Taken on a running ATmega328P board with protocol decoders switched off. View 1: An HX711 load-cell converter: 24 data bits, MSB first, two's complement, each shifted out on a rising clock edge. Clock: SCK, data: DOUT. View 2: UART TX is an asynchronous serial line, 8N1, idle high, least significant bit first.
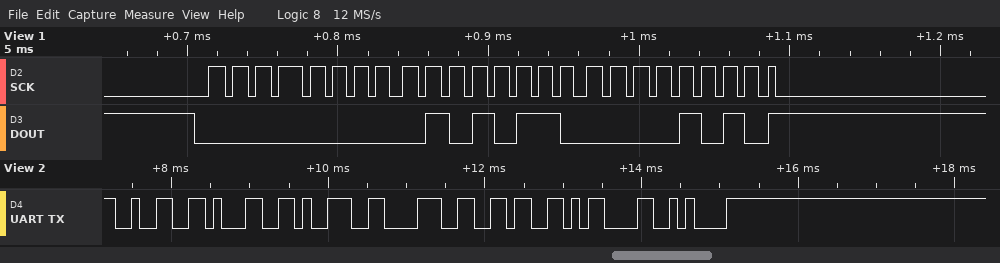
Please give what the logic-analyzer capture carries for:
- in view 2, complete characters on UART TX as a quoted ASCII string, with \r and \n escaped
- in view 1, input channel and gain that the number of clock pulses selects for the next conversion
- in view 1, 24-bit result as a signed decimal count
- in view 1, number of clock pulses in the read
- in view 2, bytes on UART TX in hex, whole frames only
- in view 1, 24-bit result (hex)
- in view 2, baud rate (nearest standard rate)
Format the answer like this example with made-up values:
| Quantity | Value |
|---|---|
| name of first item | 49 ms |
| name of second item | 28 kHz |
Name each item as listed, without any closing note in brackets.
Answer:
| Quantity | Value |
|---|---|
| in view 2, complete characters on UART TX as a quoted ASCII string, with \r and \n escaped | "21986\r\n" |
| in view 1, input channel and gain that the number of clock pulses selects for the next conversion | channel A, gain 128 |
| in view 1, 24-bit result as a signed decimal count | 22026 |
| in view 1, number of clock pulses in the read | 25 |
| in view 2, bytes on UART TX in hex, whole frames only | 32 31 39 38 36 0D 0A |
| in view 1, 24-bit result | 0x00560A |
| in view 2, baud rate | 9600 baud |
